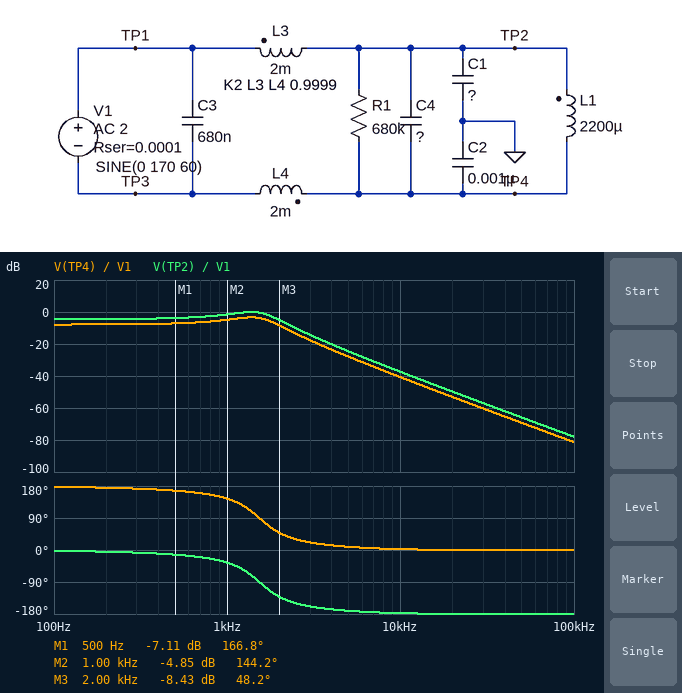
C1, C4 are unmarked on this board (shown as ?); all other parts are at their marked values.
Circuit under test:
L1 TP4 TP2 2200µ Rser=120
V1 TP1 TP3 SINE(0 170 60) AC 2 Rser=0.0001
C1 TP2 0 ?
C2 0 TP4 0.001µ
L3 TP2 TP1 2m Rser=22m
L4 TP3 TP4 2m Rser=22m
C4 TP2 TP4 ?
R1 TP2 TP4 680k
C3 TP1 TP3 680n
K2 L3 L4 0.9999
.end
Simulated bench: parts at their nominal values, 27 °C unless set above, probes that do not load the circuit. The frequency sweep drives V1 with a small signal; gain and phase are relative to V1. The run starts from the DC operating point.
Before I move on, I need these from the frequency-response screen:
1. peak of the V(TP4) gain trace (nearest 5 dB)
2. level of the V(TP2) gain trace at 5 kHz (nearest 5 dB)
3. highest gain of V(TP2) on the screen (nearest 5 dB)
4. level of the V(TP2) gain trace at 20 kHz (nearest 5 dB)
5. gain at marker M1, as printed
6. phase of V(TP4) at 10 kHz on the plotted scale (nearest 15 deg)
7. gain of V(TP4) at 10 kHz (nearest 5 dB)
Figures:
-5 dB
-25 dB
0 dB
-50 dB
-7.11 dB
0 deg
-40 dB
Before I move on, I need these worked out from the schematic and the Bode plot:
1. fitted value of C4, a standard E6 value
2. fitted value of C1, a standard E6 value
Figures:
1.5 µF
680 pF
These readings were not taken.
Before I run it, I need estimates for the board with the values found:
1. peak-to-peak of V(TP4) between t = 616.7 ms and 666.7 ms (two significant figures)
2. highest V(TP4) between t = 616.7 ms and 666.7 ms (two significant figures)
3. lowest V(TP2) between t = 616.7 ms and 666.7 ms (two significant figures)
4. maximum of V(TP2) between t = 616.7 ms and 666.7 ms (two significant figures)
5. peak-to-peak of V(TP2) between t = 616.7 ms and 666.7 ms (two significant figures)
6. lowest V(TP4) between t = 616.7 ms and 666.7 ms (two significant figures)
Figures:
140 V
69 V
-100 V
100 V
200 V
-69 V
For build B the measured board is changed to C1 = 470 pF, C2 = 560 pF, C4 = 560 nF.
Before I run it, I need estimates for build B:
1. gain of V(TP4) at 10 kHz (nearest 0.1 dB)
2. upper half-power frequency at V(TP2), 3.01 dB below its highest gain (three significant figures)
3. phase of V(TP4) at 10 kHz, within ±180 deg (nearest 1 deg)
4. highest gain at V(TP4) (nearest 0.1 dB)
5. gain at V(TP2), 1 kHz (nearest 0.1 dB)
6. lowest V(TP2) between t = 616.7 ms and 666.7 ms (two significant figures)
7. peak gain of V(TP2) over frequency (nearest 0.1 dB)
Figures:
-30.2 dB
3.32 kHz
7 deg
-6.1 dB
-5.0 dB
-92 V
-4.6 dB
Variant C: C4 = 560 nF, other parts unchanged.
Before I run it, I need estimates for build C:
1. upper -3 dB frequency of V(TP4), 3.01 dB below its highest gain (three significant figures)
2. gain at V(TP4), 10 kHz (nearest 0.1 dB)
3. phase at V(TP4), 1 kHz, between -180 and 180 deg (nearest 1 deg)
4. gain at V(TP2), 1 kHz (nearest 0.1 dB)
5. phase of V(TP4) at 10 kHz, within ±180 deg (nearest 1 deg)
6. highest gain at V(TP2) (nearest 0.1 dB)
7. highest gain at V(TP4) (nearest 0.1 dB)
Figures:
3.32 kHz
-31.2 dB
155 deg
-4.2 dB
7 deg
-3.8 dB
-7.2 dB
